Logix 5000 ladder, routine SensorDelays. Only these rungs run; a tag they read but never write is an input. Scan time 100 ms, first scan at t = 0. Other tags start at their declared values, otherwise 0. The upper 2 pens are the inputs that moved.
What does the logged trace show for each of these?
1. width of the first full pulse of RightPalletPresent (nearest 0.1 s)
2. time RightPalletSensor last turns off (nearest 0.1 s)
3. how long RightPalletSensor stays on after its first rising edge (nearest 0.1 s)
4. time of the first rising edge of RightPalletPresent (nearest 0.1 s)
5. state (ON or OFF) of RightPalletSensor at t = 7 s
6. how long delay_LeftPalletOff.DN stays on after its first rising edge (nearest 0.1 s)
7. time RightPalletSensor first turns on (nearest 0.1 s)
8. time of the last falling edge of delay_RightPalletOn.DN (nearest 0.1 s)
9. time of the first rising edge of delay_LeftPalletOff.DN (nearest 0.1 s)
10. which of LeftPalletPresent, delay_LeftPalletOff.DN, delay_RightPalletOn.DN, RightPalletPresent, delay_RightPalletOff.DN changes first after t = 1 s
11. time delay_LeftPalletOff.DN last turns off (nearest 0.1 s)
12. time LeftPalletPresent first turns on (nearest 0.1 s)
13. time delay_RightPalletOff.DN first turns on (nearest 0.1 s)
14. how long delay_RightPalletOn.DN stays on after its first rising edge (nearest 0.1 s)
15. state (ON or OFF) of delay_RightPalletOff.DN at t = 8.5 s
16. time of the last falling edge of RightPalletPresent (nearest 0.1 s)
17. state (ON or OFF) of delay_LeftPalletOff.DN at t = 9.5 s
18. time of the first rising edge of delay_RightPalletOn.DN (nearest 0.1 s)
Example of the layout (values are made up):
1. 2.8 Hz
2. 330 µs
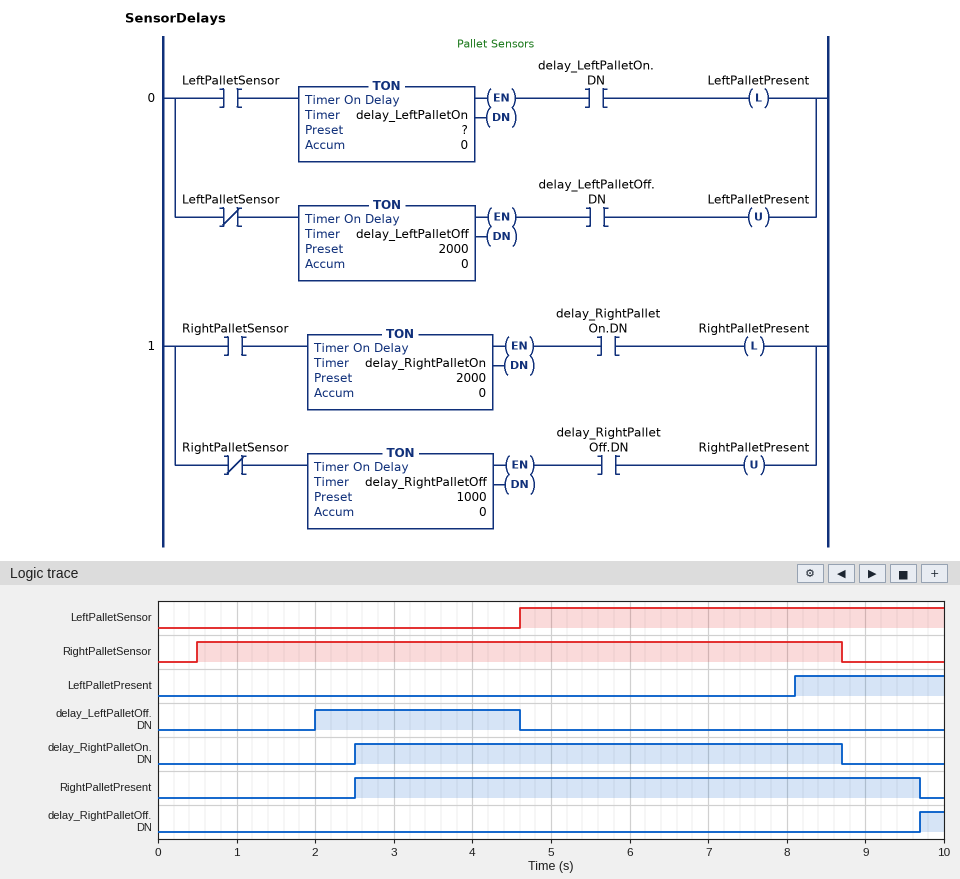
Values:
1. 7.2 s
2. 8.7 s
3. 8.2 s
4. 2.5 s
5. ON
6. 2.6 s
7. 0.5 s
8. 8.7 s
9. 2.0 s
10. delay_LeftPalletOff.DN
11. 4.6 s
12. 8.1 s
13. 9.7 s
14. 6.2 s
15. OFF
16. 9.7 s
17. OFF
18. 2.5 s
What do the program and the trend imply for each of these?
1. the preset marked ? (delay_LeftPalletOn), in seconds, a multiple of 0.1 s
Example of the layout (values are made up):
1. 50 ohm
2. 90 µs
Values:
1. 3.5 s
